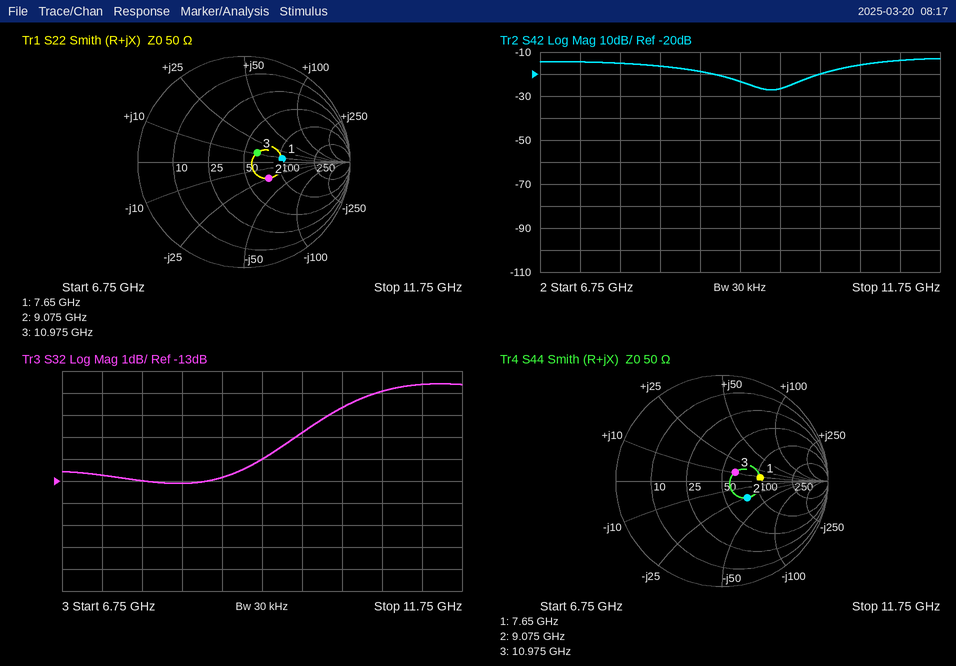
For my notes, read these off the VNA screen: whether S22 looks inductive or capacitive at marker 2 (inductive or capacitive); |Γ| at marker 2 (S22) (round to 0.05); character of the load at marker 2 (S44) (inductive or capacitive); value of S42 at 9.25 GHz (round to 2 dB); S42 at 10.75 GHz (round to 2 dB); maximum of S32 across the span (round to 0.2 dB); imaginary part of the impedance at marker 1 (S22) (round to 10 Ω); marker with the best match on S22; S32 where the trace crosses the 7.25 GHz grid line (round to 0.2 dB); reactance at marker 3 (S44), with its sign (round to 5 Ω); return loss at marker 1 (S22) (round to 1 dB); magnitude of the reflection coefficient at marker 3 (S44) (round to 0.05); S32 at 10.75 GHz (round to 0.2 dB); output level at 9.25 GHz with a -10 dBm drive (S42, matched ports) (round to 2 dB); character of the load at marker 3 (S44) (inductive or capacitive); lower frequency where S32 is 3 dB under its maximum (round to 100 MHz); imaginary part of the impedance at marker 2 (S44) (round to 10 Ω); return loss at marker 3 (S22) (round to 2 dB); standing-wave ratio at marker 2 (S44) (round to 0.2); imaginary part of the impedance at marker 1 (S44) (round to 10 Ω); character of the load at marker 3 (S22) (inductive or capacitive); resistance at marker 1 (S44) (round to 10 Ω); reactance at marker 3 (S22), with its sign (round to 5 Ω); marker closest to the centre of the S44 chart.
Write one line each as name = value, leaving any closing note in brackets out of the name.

whether S22 looks inductive or capacitive at marker 2 = capacitive
|Γ| at marker 2 (S22) = 0.30
character of the load at marker 2 (S44) = capacitive
value of S42 at 9.25 GHz = -24 dB
S42 at 10.75 GHz = -16 dB
maximum of S32 across the span = -8.6 dB
imaginary part of the impedance at marker 1 (S22) = +10 Ω
marker with the best match on S22 = marker 3
S32 where the trace crosses the 7.25 GHz grid line = -12.8 dB
reactance at marker 3 (S44), with its sign = +10 Ω
return loss at marker 1 (S22) = 9 dB
magnitude of the reflection coefficient at marker 3 (S44) = 0.15
S32 at 10.75 GHz = -9.0 dB
output level at 9.25 GHz with a -10 dBm drive (S42, matched ports) = -34 dBm
character of the load at marker 3 (S44) = inductive
lower frequency where S32 is 3 dB under its maximum = 9.4 GHz
imaginary part of the impedance at marker 2 (S44) = -30 Ω
return loss at marker 3 (S22) = 16 dB
standing-wave ratio at marker 2 (S44) = 1.8
imaginary part of the impedance at marker 1 (S44) = +10 Ω
character of the load at marker 3 (S22) = inductive
resistance at marker 1 (S44) = 110 Ω
reactance at marker 3 (S22), with its sign = +10 Ω
marker closest to the centre of the S44 chart = marker 3
